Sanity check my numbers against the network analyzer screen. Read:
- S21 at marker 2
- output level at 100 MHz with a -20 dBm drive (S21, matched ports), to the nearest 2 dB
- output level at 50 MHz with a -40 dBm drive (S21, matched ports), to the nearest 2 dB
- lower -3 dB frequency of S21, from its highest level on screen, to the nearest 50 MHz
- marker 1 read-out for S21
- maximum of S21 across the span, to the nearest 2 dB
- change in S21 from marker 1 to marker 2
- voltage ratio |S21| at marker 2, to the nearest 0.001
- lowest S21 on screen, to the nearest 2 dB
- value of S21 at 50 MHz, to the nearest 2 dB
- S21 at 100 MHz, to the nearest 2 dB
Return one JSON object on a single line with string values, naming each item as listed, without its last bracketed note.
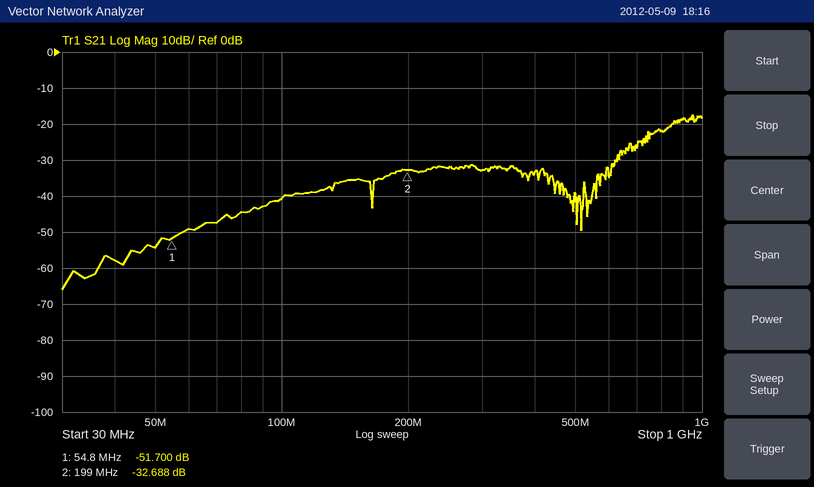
{"S21 at marker 2": "-32.688 dB", "output level at 100 MHz with a -20 dBm drive (S21, matched ports), to the nearest 2 dB": "-60 dBm", "output level at 50 MHz with a -40 dBm drive (S21, matched ports), to the nearest 2 dB": "-94 dBm", "lower -3 dB frequency of S21, from its highest level on screen, to the nearest 50 MHz": "850 MHz", "marker 1 read-out for S21": "-51.700 dB", "maximum of S21 across the span, to the nearest 2 dB": "-18 dB", "change in S21 from marker 1 to marker 2": "19.012 dB", "voltage ratio |S21| at marker 2, to the nearest 0.001": "0.023", "lowest S21 on screen, to the nearest 2 dB": "-66 dB", "value of S21 at 50 MHz, to the nearest 2 dB": "-54 dB", "S21 at 100 MHz, to the nearest 2 dB": "-40 dB"}
